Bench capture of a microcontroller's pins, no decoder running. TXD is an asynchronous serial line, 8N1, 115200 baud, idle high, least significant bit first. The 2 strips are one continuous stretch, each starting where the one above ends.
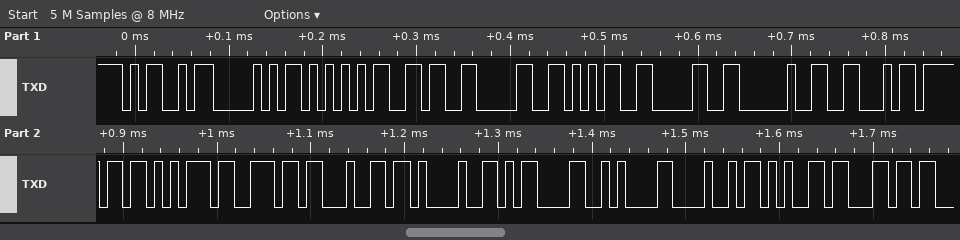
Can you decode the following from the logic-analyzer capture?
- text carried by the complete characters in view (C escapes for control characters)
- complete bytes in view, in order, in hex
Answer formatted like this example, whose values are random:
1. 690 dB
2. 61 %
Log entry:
1. "MPU6050 Found!\r\nHel"
2. 4D 50 55 36 30 35 30 20 46 6F 75 6E 64 21 0D 0A 48 65 6C
